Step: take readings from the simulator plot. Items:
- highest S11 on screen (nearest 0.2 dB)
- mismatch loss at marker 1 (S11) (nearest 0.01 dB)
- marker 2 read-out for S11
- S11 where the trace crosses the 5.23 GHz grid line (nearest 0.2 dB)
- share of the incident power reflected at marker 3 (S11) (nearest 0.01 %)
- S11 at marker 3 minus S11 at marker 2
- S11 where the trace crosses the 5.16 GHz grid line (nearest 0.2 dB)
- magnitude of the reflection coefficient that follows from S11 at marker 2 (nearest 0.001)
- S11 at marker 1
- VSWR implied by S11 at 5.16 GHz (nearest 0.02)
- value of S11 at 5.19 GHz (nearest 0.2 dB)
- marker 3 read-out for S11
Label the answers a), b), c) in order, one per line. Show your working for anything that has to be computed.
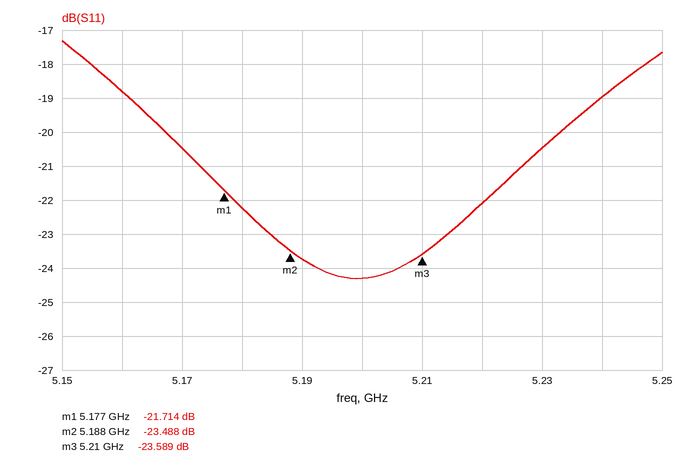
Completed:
a) -17.4 dB
b) −10 log10(1 − 10^(-21.714/10)) ≈ 0.03 dB
c) -23.488 dB
d) -20.4 dB
e) 10^(-23.589/10) ≈ 0.44 %
f) -23.589 − (-23.488) = -0.101 dB
g) -18.8 dB
h) 10^(-23.488/20) ≈ 0.067
i) -21.714 dB
j) |Γ| = 10^(-18.8/20) = 0.1148; VSWR = (1 + 0.1148)/(1 − 0.1148) ≈ 1.26
k) -23.8 dB
l) -23.589 dB
